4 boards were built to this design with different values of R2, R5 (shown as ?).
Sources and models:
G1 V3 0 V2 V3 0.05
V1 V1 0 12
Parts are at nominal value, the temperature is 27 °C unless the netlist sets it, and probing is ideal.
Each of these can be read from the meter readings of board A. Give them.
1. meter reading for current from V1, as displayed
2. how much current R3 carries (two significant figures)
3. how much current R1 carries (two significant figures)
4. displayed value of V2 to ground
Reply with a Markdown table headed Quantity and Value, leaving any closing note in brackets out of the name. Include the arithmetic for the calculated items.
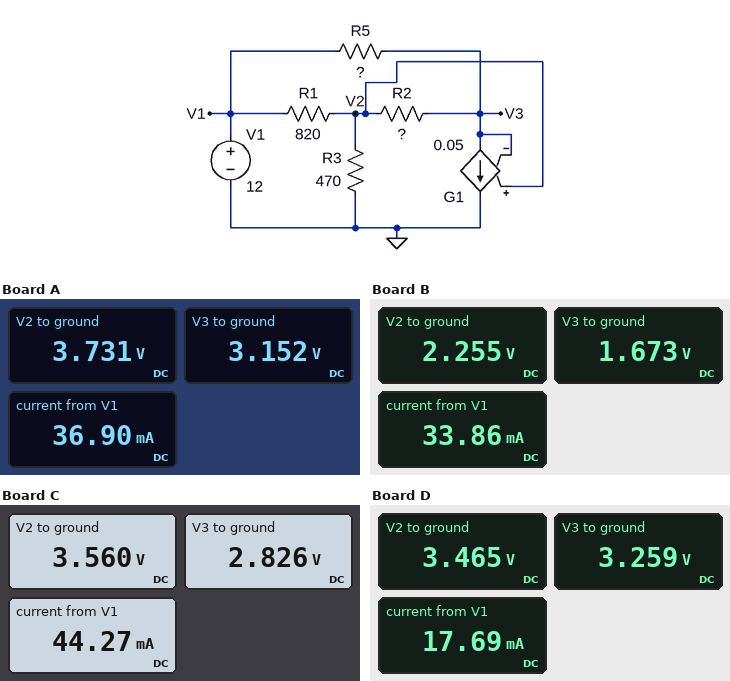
| Quantity | Value |
|---|---|
| meter reading for current from V1, as displayed | 36.90 mA |
| how much current R3 carries | (3.731 V) / 470 Ω = 7.9 mA |
| how much current R1 carries | (12 V - 3.731 V) / 820 Ω = 10 mA |
| displayed value of V2 to ground | 3.731 V |
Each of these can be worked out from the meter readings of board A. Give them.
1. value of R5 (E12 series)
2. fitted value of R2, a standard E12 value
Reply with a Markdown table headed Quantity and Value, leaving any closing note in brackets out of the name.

| Quantity | Value |
|---|---|
| value of R5 | 330 Ω |
| fitted value of R2, a standard E12 value | 270 Ω |
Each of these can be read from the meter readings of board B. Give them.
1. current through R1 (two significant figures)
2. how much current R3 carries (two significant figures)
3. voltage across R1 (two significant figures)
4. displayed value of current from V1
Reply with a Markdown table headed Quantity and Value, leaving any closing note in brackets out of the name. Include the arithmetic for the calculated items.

| Quantity | Value |
|---|---|
| current through R1 | (12 V - 2.255 V) / 820 Ω = 12 mA |
| how much current R3 carries | (2.255 V) / 470 Ω = 4.8 mA |
| voltage across R1 | 12 V - 2.255 V = 9.7 V |
| displayed value of current from V1 | 33.86 mA |
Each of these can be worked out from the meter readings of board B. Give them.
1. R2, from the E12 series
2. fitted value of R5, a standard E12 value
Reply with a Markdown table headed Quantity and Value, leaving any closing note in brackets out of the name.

| Quantity | Value |
|---|---|
| R2, from the E12 series | 82 Ω |
| fitted value of R5, a standard E12 value | 470 Ω |
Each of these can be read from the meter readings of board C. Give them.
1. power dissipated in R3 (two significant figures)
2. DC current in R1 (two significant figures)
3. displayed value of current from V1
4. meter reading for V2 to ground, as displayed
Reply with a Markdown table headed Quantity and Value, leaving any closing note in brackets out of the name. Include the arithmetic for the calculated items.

| Quantity | Value |
|---|---|
| power dissipated in R3 | (3.56 V)^2 / 470 Ω = 27 mW |
| DC current in R1 | (12 V - 3.56 V) / 820 Ω = 10 mA |
| displayed value of current from V1 | 44.27 mA |
| meter reading for V2 to ground, as displayed | 3.560 V |
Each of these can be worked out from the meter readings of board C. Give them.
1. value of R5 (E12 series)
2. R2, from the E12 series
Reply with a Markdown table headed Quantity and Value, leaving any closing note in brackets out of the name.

| Quantity | Value |
|---|---|
| value of R5 | 270 Ω |
| R2, from the E12 series | 270 Ω |
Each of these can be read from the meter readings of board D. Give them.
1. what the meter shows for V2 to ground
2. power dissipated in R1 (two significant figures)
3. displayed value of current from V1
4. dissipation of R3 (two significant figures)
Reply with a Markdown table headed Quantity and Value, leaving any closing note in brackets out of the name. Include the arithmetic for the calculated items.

| Quantity | Value |
|---|---|
| what the meter shows for V2 to ground | 3.465 V |
| power dissipated in R1 | (12 V - 3.465 V)^2 / 820 Ω = 89 mW |
| displayed value of current from V1 | 17.69 mA |
| dissipation of R3 | (3.465 V)^2 / 470 Ω = 26 mW |
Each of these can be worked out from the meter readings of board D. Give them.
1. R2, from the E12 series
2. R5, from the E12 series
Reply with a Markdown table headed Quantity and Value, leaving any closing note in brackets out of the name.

| Quantity | Value |
|---|---|
| R2, from the E12 series | 68 Ω |
| R5, from the E12 series | 1.2 kΩ |
